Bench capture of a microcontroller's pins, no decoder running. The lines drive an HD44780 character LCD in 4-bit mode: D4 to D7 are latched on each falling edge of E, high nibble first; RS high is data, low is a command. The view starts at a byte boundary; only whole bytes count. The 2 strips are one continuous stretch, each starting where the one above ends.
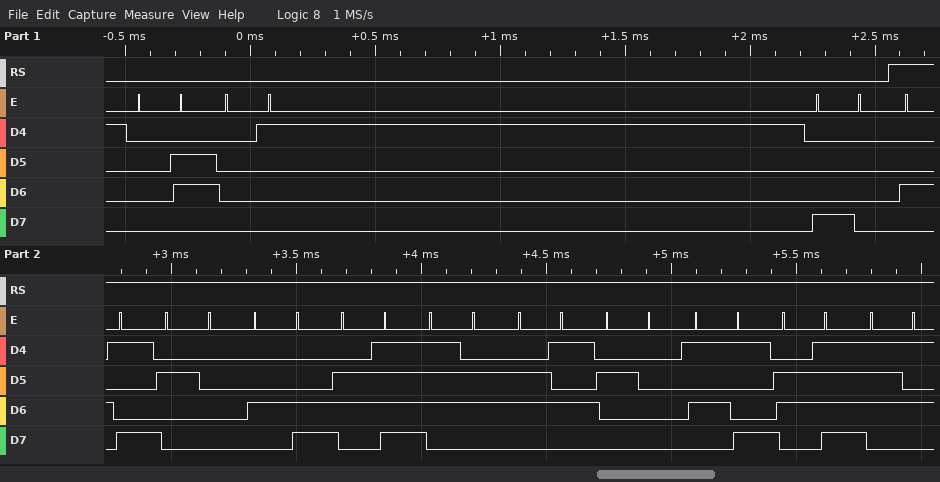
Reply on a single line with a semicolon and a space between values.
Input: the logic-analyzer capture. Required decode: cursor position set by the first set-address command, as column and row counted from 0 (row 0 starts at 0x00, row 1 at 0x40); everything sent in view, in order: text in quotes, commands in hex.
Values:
column 0, row 0; 0x06 0x01 0x80 "I Love You"
